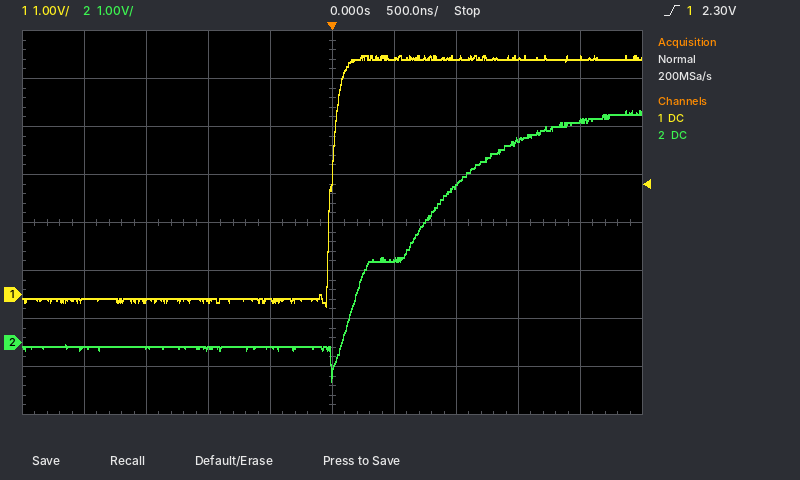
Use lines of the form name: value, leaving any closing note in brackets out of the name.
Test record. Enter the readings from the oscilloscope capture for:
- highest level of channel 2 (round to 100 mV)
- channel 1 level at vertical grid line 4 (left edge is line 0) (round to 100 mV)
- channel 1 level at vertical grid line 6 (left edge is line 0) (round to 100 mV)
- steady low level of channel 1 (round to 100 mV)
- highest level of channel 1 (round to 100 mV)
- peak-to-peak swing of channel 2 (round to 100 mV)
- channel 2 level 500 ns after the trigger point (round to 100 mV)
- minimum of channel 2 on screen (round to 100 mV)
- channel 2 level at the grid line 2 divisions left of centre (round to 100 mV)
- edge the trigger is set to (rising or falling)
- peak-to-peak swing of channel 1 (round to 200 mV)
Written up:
highest level of channel 2: 4.8 V
channel 1 level at vertical grid line 4 (left edge is line 0): -100 mV
channel 1 level at vertical grid line 6 (left edge is line 0): 4.9 V
steady low level of channel 1: -100 mV
highest level of channel 1: 5.0 V
peak-to-peak swing of channel 2: 5.6 V
channel 2 level 500 ns after the trigger point: 1.7 V
minimum of channel 2 on screen: -800 mV
channel 2 level at the grid line 2 divisions left of centre: -100 mV
edge the trigger is set to: rising
peak-to-peak swing of channel 1: 5.2 V
